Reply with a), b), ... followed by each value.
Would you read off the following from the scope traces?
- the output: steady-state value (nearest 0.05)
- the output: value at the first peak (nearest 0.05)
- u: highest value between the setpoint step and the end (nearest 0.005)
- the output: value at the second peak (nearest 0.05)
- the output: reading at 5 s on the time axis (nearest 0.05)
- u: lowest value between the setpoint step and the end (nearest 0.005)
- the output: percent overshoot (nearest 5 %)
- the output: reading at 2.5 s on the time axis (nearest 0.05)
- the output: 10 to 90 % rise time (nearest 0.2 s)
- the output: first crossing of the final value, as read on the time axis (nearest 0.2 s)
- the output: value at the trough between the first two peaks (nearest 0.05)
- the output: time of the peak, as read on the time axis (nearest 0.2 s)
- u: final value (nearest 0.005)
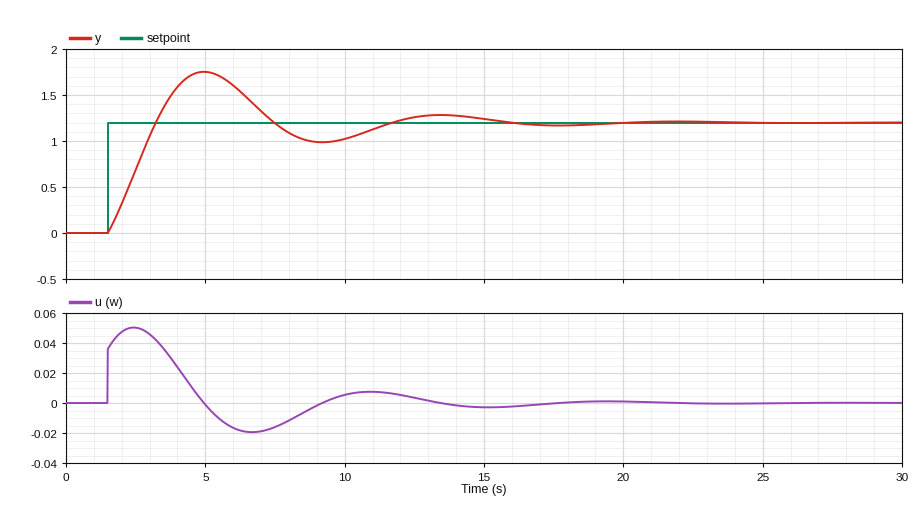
a) 1.20
b) 1.75
c) 0.050
d) 1.30
e) 1.75
f) -0.020
g) 45 %
h) 0.70
i) 1.4 s
j) 3.2 s
k) 1.00
l) 5.0 s
m) 0.000
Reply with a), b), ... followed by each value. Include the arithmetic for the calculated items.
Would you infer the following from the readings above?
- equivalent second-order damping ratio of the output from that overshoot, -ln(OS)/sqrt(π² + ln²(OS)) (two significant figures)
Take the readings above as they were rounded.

a) ln(0.45) = -0.799; 0.799 / sqrt(9.870 + 0.638) = 0.25
